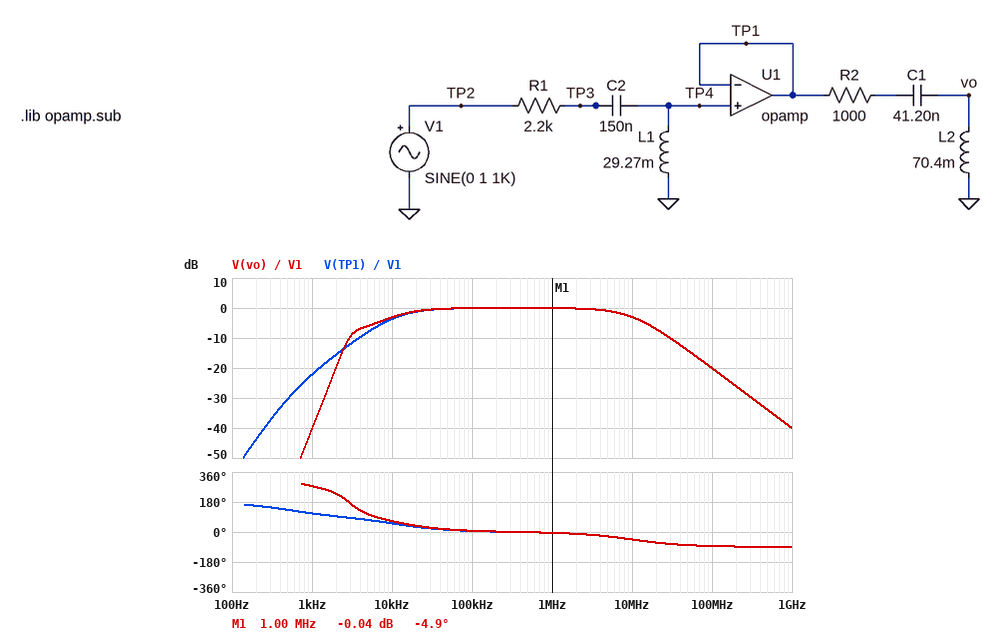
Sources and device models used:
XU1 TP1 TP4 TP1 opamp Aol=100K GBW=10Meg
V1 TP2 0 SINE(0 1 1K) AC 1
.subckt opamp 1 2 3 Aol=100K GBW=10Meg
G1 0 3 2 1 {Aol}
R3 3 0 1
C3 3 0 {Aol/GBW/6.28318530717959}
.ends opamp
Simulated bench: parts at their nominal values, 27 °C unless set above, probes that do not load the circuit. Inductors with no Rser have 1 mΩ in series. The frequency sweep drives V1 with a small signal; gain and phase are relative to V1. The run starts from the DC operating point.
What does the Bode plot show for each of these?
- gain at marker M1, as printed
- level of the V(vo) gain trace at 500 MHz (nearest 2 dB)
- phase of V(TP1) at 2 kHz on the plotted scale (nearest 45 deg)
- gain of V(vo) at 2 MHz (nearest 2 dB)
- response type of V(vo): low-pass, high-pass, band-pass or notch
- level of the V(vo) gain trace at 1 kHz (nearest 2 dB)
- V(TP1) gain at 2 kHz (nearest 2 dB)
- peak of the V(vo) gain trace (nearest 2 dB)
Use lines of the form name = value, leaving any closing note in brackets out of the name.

gain at marker M1, as printed = -0.04 dB
level of the V(vo) gain trace at 500 MHz = -34 dB
phase of V(TP1) at 2 kHz on the plotted scale = 90 deg
gain of V(vo) at 2 MHz = 0 dB
response type of V(vo): low-pass, high-pass, band-pass or notch = band-pass
level of the V(vo) gain trace at 1 kHz = -40 dB
V(TP1) gain at 2 kHz = -16 dB
peak of the V(vo) gain trace = 0 dB
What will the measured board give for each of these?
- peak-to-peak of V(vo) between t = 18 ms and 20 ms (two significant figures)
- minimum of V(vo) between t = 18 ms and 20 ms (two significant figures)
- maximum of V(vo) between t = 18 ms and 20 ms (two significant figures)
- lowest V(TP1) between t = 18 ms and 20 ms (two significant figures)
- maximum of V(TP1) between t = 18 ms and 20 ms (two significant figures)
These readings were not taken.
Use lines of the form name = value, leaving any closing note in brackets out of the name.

peak-to-peak of V(vo) between t = 18 ms and 20 ms = 19 mV
minimum of V(vo) between t = 18 ms and 20 ms = -9.6 mV
maximum of V(vo) between t = 18 ms and 20 ms = 9.6 mV
lowest V(TP1) between t = 18 ms and 20 ms = -78 mV
maximum of V(TP1) between t = 18 ms and 20 ms = 78 mV
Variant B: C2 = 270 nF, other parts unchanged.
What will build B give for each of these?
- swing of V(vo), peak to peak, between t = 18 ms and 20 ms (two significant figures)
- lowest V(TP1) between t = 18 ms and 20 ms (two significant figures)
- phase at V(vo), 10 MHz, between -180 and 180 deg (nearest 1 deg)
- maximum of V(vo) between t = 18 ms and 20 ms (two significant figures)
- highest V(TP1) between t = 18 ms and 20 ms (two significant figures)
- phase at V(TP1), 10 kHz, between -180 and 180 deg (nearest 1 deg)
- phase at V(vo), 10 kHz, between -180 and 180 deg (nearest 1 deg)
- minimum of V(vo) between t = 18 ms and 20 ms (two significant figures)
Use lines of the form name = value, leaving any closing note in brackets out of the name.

swing of V(vo), peak to peak, between t = 18 ms and 20 ms = 20 mV
lowest V(TP1) between t = 18 ms and 20 ms = -82 mV
phase at V(vo), 10 MHz, between -180 and 180 deg = -45 deg
maximum of V(vo) between t = 18 ms and 20 ms = 10 mV
highest V(TP1) between t = 18 ms and 20 ms = 82 mV
phase at V(TP1), 10 kHz, between -180 and 180 deg = 51 deg
phase at V(vo), 10 kHz, between -180 and 180 deg = 65 deg
minimum of V(vo) between t = 18 ms and 20 ms = -10 mV
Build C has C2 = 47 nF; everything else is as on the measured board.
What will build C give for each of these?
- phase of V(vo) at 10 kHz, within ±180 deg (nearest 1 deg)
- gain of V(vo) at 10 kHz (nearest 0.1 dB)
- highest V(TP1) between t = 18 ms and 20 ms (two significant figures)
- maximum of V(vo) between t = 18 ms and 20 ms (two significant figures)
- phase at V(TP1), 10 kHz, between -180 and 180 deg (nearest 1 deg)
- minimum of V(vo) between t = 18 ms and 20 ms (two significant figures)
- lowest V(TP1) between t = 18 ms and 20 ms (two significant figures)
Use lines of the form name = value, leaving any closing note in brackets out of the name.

phase of V(vo) at 10 kHz, within ±180 deg = 70 deg
gain of V(vo) at 10 kHz = -2.7 dB
highest V(TP1) between t = 18 ms and 20 ms = 47 mV
maximum of V(vo) between t = 18 ms and 20 ms = 5.9 mV
phase at V(TP1), 10 kHz, between -180 and 180 deg = 56 deg
minimum of V(vo) between t = 18 ms and 20 ms = -5.9 mV
lowest V(TP1) between t = 18 ms and 20 ms = -47 mV
